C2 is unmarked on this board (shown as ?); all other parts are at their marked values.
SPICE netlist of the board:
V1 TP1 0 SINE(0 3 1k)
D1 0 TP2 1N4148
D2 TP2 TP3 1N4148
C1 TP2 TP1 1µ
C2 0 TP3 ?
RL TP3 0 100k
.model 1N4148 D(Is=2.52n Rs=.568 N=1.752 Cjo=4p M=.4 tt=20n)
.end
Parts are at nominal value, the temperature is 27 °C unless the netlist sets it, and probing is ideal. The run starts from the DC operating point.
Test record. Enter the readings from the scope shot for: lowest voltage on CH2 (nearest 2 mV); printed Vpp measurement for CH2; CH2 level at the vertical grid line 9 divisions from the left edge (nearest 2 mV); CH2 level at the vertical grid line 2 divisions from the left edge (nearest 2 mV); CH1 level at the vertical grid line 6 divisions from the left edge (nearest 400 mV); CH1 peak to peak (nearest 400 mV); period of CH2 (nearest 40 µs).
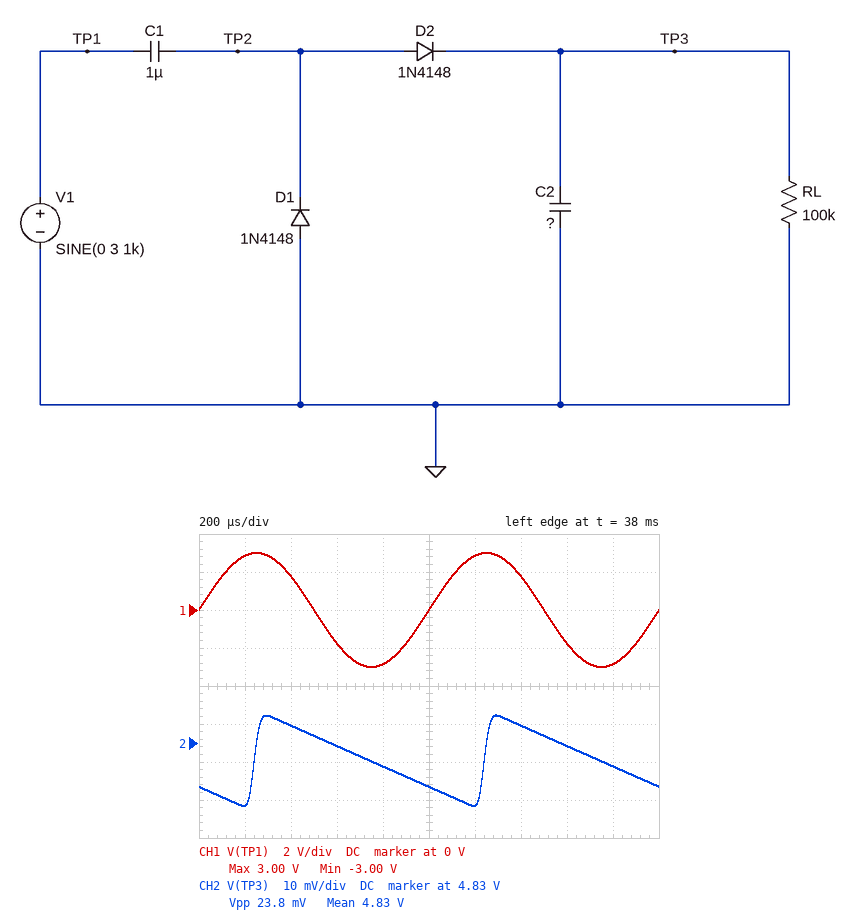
4.814 V
23.8 mV
4.824 V
4.834 V
2.8 V
6.0 V
1.00 ms
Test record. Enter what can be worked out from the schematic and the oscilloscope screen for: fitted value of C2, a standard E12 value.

1.8 µF
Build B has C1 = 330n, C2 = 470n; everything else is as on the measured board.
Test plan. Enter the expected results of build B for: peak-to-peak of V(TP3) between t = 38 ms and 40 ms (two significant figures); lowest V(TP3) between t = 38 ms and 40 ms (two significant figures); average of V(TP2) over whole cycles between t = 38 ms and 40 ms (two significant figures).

89 mV
4.7 V
2.4 V
